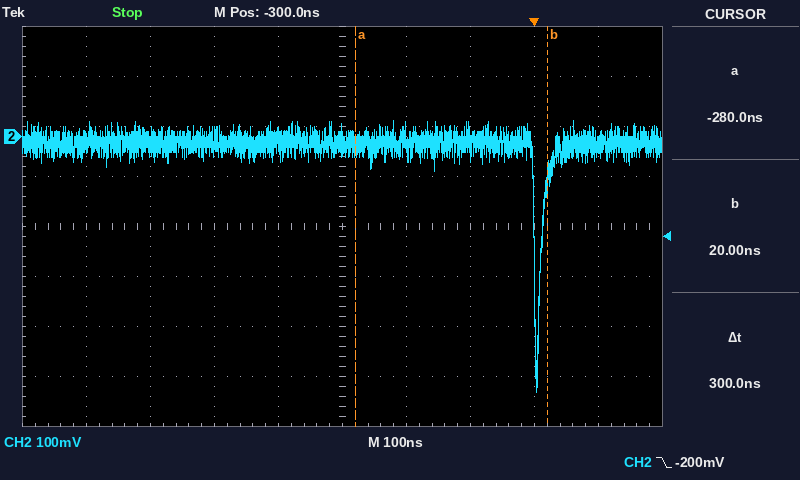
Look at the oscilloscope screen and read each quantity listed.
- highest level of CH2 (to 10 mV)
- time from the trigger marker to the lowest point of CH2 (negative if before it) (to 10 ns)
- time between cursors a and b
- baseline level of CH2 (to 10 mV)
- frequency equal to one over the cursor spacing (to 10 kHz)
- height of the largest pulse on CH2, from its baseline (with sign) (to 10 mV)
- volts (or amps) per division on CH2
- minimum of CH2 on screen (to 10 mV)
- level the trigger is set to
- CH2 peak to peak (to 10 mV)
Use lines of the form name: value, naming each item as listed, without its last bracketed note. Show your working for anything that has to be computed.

highest level of CH2: 30 mV
time from the trigger marker to the lowest point of CH2 (negative if before it): 0 ns
time between cursors a and b: 300 ns
baseline level of CH2: -10 mV
frequency equal to one over the cursor spacing: 1 / 300 ns ≈ 3.33 MHz
height of the largest pulse on CH2, from its baseline (with sign): -510 mV − (-10 mV) = -500 mV
volts (or amps) per division on CH2: 100 mV
minimum of CH2 on screen: -510 mV
level the trigger is set to: -200 mV
CH2 peak to peak: 30 mV − (-510 mV) = 540 mV
